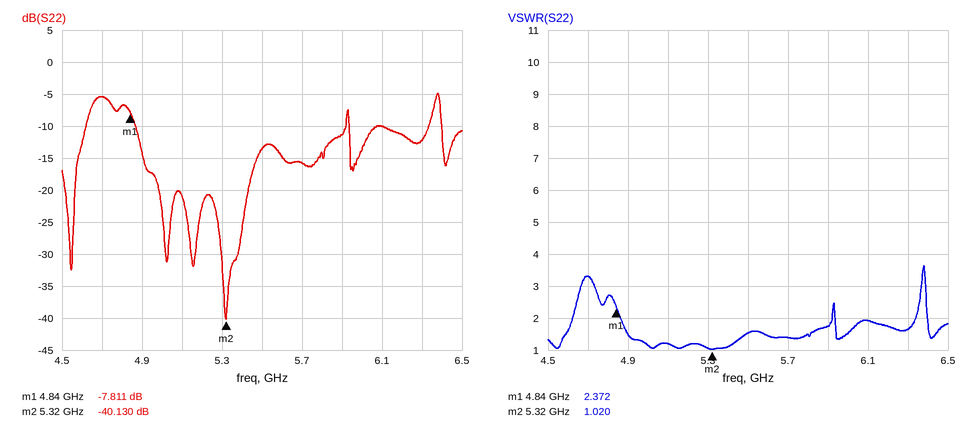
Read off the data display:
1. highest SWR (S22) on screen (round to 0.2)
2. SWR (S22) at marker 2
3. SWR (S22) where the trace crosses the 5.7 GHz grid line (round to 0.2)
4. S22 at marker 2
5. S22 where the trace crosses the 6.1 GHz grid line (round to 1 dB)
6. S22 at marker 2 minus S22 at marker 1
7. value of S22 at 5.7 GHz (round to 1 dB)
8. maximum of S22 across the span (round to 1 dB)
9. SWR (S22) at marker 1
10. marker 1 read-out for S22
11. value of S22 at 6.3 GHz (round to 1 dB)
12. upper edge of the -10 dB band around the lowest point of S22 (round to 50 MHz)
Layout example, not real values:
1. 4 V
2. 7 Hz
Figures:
1. 3.6
2. 1.020
3. 1.4
4. -40.130 dB
5. -10 dB
6. -32.319 dB
7. -16 dB
8. -5 dB
9. 2.372
10. -7.811 dB
11. -12 dB
12. 5.90 GHz
